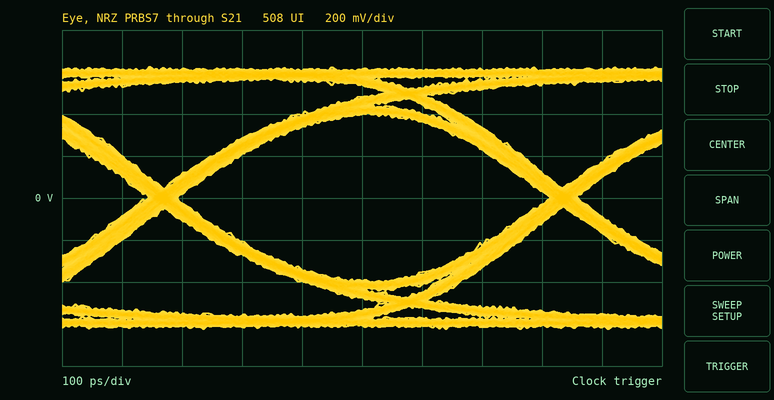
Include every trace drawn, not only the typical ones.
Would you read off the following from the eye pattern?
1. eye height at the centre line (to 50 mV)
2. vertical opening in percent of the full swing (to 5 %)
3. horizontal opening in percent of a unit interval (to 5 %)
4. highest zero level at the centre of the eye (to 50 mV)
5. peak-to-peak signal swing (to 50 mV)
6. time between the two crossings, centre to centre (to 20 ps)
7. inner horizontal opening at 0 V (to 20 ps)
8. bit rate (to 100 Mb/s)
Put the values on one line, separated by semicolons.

800 mV; 65 %; 95 %; -400 mV; 1.25 V; 660 ps; 620 ps; 1.5 Gb/s
